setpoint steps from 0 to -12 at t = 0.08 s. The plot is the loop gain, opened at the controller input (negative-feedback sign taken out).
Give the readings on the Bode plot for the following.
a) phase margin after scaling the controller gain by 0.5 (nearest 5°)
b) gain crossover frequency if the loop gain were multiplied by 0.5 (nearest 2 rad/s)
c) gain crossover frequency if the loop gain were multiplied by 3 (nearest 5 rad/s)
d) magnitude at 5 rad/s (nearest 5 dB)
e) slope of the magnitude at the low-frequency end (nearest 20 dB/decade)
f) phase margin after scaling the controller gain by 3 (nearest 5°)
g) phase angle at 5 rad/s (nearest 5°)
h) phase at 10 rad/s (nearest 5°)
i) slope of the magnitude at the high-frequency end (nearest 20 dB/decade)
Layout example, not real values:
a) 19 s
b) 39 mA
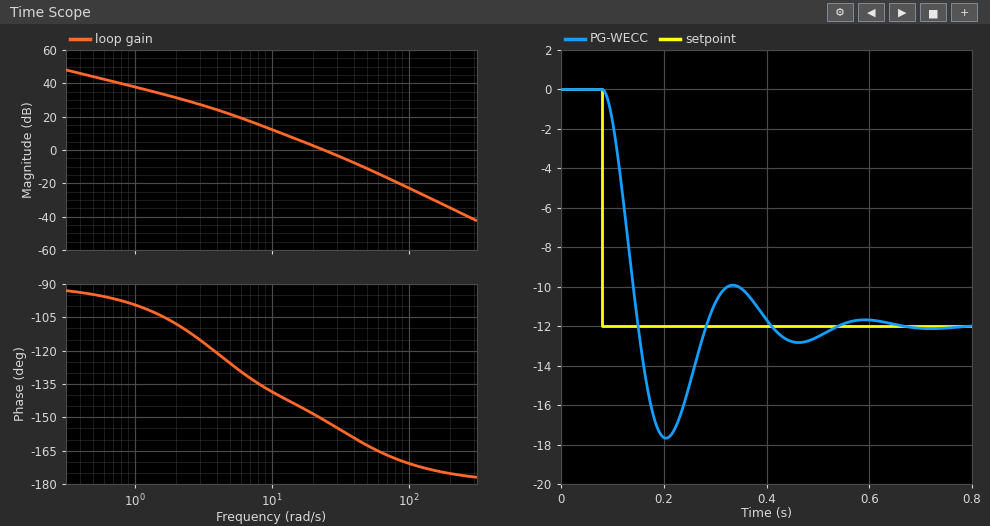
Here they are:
a) 35°
b) 16 rad/s
c) 45 rad/s
d) 20 dB
e) -20 dB/decade
f) 20°
g) -125°
h) -140°
i) -40 dB/decade
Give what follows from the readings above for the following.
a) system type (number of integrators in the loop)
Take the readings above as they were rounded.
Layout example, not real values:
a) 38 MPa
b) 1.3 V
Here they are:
a) 1
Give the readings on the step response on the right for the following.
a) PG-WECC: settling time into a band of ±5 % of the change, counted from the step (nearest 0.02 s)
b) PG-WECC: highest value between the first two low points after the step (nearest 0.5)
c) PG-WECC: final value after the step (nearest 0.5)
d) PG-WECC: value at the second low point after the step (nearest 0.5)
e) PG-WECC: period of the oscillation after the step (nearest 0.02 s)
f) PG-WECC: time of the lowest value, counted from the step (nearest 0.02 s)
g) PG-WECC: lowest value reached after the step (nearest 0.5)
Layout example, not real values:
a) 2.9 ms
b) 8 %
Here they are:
a) 0.42 s
b) -10.0
c) -12.0
d) -13.0
e) 0.26 s
f) 0.12 s
g) -17.5
